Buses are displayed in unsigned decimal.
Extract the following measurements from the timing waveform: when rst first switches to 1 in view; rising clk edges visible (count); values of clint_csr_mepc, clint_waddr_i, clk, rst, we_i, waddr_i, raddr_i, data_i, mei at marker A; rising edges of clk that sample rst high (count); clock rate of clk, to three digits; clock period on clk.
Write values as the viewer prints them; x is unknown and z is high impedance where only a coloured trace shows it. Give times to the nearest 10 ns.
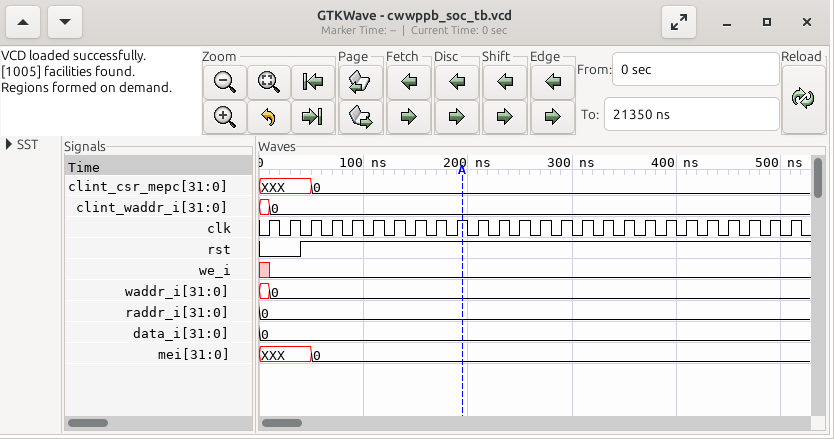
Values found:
40 ns
26
clint_csr_mepc=0, clint_waddr_i=0, clk=1, rst=1, we_i=0, waddr_i=0, raddr_i=0, data_i=0, mei=0
24
50.0 MHz
20 ns
